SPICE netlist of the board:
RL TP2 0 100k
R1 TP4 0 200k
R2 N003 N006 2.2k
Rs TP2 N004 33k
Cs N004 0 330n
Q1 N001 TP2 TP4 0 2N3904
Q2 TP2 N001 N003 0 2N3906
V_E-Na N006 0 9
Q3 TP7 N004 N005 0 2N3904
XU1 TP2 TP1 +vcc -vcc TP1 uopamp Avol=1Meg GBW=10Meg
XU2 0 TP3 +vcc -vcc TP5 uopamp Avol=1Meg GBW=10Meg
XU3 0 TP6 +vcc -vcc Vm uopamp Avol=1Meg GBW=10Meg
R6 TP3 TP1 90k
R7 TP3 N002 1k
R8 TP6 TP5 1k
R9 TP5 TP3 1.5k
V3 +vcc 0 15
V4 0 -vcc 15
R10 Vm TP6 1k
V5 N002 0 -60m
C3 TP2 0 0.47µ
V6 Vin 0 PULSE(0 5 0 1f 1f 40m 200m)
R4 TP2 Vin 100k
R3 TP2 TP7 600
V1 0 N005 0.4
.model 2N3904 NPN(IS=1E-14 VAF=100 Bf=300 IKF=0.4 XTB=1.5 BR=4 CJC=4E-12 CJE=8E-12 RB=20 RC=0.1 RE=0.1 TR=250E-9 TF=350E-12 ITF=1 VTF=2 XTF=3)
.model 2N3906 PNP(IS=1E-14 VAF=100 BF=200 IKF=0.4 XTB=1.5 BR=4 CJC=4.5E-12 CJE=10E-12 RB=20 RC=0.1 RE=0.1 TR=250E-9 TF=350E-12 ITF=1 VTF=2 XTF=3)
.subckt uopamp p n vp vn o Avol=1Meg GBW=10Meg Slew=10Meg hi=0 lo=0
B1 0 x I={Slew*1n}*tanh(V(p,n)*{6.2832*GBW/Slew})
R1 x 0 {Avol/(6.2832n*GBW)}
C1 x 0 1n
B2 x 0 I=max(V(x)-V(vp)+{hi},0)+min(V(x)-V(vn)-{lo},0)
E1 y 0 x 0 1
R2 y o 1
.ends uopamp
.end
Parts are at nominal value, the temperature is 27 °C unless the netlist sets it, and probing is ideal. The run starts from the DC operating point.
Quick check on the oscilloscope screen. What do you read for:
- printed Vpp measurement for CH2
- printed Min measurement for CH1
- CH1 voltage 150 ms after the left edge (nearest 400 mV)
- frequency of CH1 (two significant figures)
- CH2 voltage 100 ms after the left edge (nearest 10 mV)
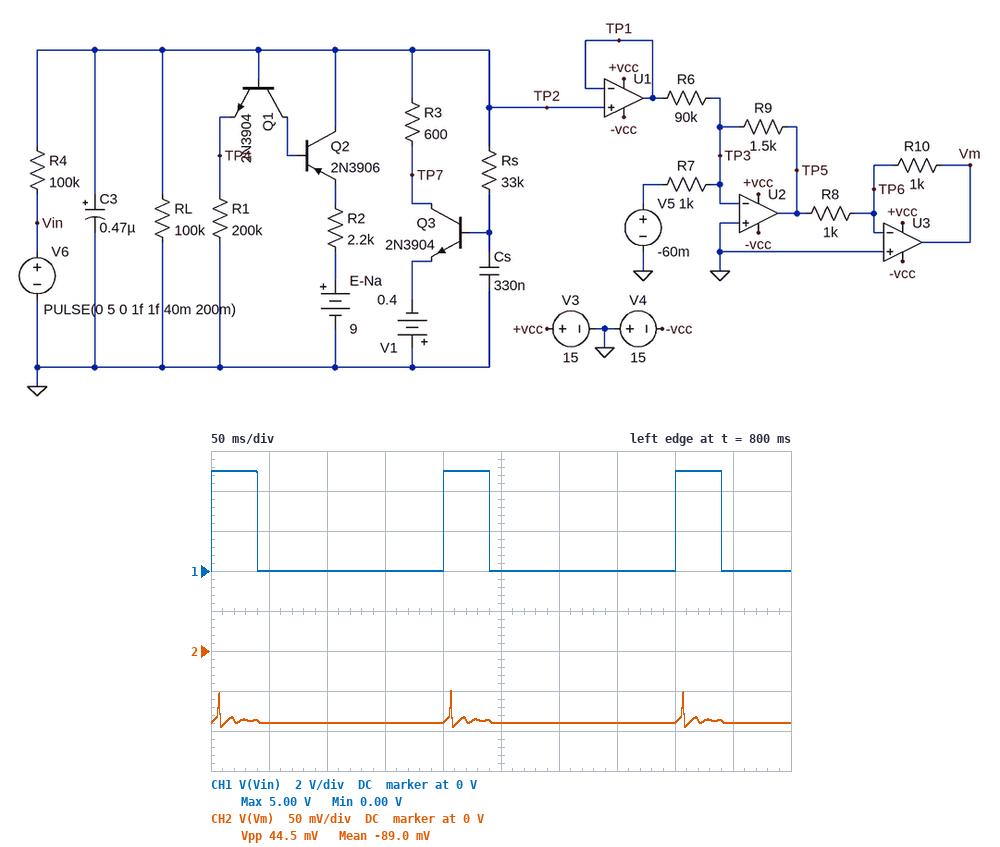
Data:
44.5 mV
0.00 V
0 V
5.0 Hz
-90 mV
